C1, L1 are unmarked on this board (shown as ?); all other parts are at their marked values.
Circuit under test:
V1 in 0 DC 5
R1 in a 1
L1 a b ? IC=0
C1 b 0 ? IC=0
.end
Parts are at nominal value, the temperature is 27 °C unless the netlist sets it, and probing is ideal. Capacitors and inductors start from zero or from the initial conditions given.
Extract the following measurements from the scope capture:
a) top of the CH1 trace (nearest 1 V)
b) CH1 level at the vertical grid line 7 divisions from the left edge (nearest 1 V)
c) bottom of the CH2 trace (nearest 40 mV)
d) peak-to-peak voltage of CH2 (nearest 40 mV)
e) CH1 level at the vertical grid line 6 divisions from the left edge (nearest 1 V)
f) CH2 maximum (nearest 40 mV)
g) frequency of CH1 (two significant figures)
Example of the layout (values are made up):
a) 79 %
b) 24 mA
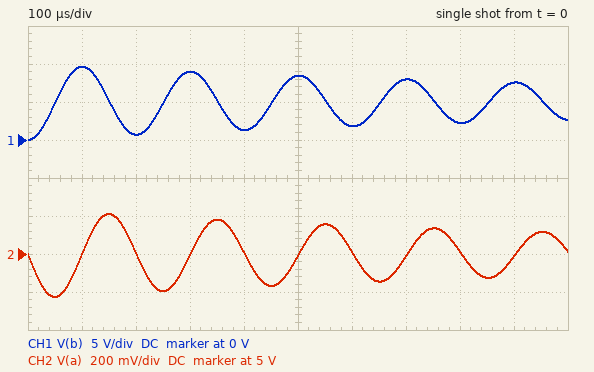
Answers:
a) 10 V
b) 8 V
c) 4.76 V
d) 440 mV
e) 2 V
f) 5.20 V
g) 5.0 kHz
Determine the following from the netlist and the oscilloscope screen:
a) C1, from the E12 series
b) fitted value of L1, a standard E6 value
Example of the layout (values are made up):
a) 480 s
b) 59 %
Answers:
a) 1.5 µF
b) 680 µH
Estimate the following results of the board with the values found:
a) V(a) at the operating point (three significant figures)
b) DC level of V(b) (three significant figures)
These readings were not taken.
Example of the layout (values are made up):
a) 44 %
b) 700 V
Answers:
a) 5.00 V
b) 5.00 V
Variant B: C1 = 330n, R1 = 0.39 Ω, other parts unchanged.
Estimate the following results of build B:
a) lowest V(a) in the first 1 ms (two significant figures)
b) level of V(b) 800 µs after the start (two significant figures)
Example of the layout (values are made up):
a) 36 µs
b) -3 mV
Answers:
a) 5.0 V
b) 9.0 V
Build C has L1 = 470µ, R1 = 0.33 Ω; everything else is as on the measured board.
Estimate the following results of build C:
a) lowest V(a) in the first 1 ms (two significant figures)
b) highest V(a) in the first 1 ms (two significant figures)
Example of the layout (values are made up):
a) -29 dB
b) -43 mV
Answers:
a) 4.9 V
b) 5.1 V
